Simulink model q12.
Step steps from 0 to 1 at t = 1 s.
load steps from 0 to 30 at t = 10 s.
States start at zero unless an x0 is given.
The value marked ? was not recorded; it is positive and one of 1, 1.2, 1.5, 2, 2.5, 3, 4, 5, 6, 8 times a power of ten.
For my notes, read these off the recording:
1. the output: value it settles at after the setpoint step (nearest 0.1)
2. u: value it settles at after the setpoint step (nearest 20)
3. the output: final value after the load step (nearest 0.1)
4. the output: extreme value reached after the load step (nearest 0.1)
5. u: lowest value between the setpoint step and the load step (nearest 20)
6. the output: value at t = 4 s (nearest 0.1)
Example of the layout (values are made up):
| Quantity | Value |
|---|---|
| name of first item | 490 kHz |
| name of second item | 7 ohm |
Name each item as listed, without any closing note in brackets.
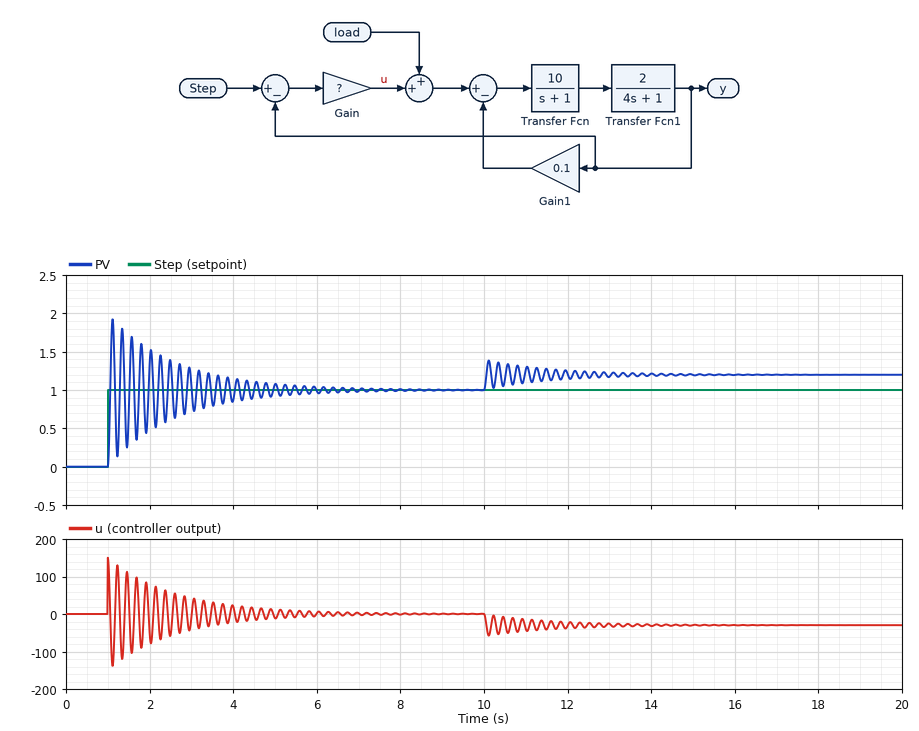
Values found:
| Quantity | Value |
|---|---|
| the output: value it settles at after the setpoint step | 1.0 |
| u: value it settles at after the setpoint step | 0 |
| the output: final value after the load step | 1.2 |
| the output: extreme value reached after the load step | 1.4 |
| u: lowest value between the setpoint step and the load step | -140 |
| the output: value at t = 4 s | 0.9 |
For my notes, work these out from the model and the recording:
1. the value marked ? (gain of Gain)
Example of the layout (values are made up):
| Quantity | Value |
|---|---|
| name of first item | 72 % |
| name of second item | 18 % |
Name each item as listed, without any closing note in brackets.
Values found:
| Quantity | Value |
|---|---|
| the value marked ? | 150 |
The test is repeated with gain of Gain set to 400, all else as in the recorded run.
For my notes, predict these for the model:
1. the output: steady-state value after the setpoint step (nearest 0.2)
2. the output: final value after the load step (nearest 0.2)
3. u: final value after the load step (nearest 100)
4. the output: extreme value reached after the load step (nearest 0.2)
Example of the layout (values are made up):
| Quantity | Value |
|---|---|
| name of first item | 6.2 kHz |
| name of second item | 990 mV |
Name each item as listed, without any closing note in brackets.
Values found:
| Quantity | Value |
|---|---|
| the output: steady-state value after the setpoint step | 1.0 |
| the output: final value after the load step | 1.0 |
| u: final value after the load step | 0 |
| the output: extreme value reached after the load step | 1.2 |
